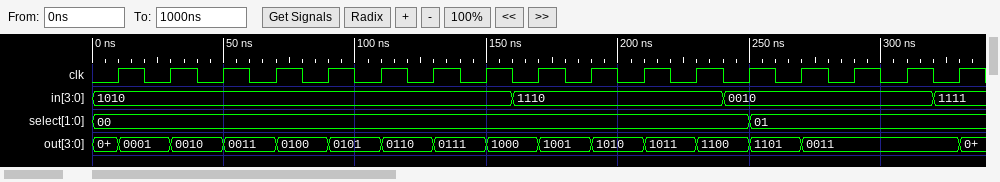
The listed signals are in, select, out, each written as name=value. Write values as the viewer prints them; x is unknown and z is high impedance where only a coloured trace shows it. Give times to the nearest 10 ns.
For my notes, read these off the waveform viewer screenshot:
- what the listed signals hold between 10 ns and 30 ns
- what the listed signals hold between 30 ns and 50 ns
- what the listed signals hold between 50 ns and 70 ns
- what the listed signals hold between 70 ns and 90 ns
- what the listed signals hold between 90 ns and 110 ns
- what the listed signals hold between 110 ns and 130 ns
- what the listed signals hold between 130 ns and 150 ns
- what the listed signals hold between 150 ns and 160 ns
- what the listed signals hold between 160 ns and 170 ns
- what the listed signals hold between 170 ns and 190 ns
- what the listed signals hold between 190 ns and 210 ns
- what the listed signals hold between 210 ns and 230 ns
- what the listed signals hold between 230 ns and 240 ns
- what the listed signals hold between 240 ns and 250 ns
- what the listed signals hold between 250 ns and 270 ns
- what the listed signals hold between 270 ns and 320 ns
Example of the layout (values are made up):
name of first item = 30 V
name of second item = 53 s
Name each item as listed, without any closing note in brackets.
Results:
what the listed signals hold between 10 ns and 30 ns = in=1010, select=00, out=0001
what the listed signals hold between 30 ns and 50 ns = in=1010, select=00, out=0010
what the listed signals hold between 50 ns and 70 ns = in=1010, select=00, out=0011
what the listed signals hold between 70 ns and 90 ns = in=1010, select=00, out=0100
what the listed signals hold between 90 ns and 110 ns = in=1010, select=00, out=0101
what the listed signals hold between 110 ns and 130 ns = in=1010, select=00, out=0110
what the listed signals hold between 130 ns and 150 ns = in=1010, select=00, out=0111
what the listed signals hold between 150 ns and 160 ns = in=1010, select=00, out=1000
what the listed signals hold between 160 ns and 170 ns = in=1110, select=00, out=1000
what the listed signals hold between 170 ns and 190 ns = in=1110, select=00, out=1001
what the listed signals hold between 190 ns and 210 ns = in=1110, select=00, out=1010
what the listed signals hold between 210 ns and 230 ns = in=1110, select=00, out=1011
what the listed signals hold between 230 ns and 240 ns = in=1110, select=00, out=1100
what the listed signals hold between 240 ns and 250 ns = in=0010, select=00, out=1100
what the listed signals hold between 250 ns and 270 ns = in=0010, select=01, out=1101
what the listed signals hold between 270 ns and 320 ns = in=0010, select=01, out=0011
